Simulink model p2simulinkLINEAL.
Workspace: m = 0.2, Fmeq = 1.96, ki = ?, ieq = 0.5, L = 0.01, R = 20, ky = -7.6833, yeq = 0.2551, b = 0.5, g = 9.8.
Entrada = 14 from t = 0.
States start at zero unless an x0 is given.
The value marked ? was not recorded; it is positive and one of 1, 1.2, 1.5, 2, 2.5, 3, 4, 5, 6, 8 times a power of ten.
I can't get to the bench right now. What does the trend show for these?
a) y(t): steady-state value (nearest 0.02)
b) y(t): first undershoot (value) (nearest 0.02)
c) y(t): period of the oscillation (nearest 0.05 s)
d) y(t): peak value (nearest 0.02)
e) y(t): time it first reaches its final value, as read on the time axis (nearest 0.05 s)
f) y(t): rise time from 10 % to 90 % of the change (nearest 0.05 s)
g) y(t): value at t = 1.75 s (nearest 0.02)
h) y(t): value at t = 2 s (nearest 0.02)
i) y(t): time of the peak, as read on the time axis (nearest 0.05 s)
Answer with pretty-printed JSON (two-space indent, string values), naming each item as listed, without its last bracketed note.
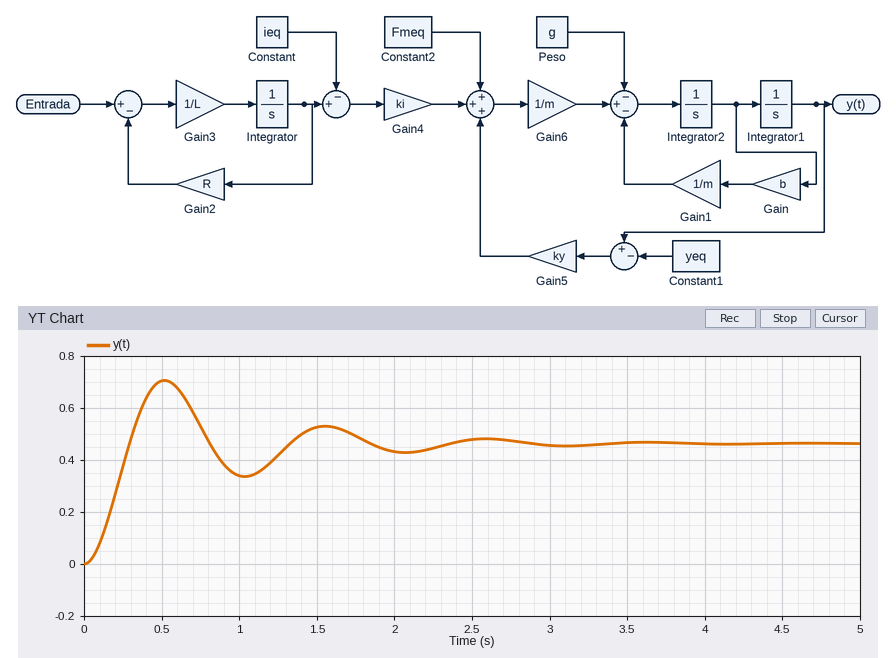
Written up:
{
  "y(t): steady-state value": "0.46",
  "y(t): first undershoot (value)": "0.34",
  "y(t): period of the oscillation": "1.05 s",
  "y(t): peak value": "0.70",
  "y(t): time it first reaches its final value, as read on the time axis": "0.30 s",
  "y(t): rise time from 10 % to 90 % of the change": "0.20 s",
  "y(t): value at t = 1.75 s": "0.50",
  "y(t): value at t = 2 s": "0.44",
  "y(t): time of the peak, as read on the time axis": "0.50 s"
}
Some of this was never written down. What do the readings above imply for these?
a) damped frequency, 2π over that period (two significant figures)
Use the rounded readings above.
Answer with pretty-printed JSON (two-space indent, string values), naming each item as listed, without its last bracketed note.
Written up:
{
  "damped frequency, 2π over that period": "6.0 rad/s"
}
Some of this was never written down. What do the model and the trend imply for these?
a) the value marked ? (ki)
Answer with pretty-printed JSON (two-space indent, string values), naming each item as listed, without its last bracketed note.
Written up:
{
  "the value marked ?": "8"
}
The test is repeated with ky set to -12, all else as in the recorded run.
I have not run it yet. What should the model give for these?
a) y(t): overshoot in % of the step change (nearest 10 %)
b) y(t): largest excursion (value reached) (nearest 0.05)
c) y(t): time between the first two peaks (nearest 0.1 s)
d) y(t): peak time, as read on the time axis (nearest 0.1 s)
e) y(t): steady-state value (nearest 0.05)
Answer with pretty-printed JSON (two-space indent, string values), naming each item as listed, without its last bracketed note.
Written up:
{
  "y(t): overshoot in % of the step change": "60 %",
  "y(t): largest excursion (value reached)": "0.60",
  "y(t): time between the first two peaks": "0.8 s",
  "y(t): peak time, as read on the time axis": "0.4 s",
  "y(t): steady-state value": "0.40"
}
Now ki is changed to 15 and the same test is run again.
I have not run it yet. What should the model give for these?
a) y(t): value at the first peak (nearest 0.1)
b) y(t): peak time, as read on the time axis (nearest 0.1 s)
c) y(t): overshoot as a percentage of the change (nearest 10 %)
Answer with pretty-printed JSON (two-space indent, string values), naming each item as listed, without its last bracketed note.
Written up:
{
  "y(t): value at the first peak": "1.0",
  "y(t): peak time, as read on the time axis": "0.5 s",
  "y(t): overshoot as a percentage of the change": "50 %"
}
